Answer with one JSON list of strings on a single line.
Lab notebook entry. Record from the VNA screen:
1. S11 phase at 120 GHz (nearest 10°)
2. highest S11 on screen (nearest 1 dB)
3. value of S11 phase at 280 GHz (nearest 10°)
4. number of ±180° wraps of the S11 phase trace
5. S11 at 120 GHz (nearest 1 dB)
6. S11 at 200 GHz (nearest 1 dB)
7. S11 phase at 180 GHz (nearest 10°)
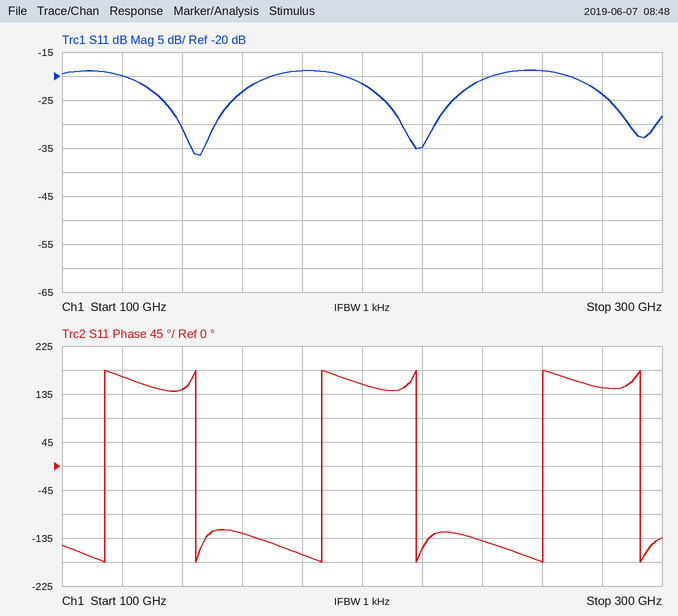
["170°", "-19 dB", "150°", "6", "-20 dB", "-22 dB", "-170°"]
